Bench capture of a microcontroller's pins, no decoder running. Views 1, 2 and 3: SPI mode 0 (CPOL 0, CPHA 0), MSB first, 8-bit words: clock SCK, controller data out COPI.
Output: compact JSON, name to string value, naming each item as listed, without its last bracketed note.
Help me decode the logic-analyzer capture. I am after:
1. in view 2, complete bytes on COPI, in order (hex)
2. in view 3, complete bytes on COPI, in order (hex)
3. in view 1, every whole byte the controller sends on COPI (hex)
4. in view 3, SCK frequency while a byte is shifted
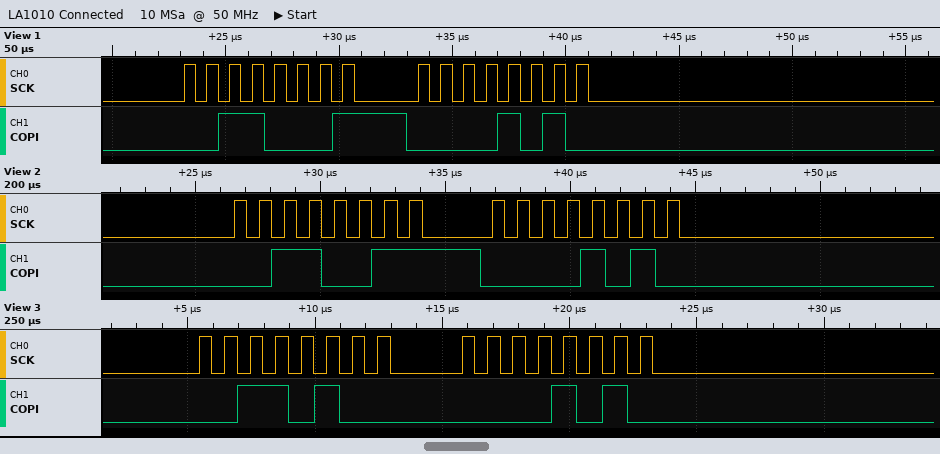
{"in view 2, complete bytes on COPI, in order": "33 0A", "in view 3, complete bytes on COPI, in order": "34 0A", "in view 1, every whole byte the controller sends on COPI": "31 0A", "in view 3, SCK frequency while a byte is shifted": "1 MHz"}
